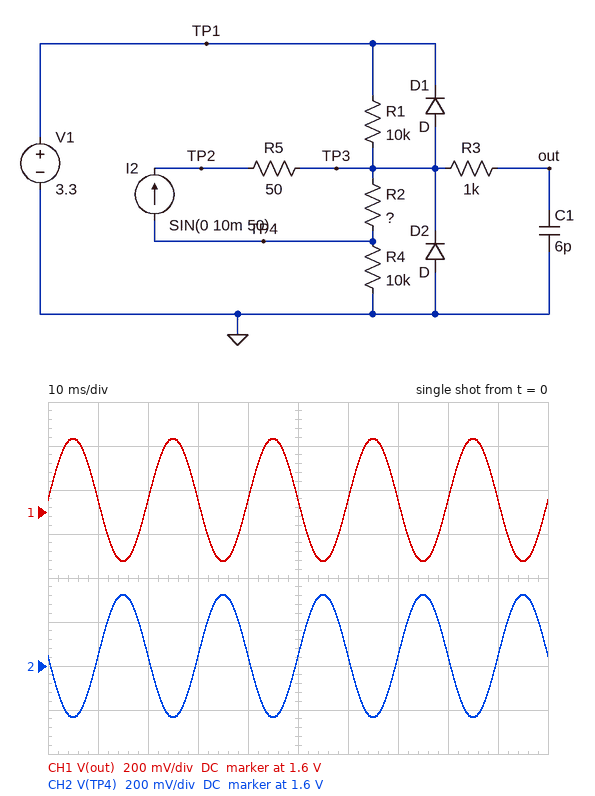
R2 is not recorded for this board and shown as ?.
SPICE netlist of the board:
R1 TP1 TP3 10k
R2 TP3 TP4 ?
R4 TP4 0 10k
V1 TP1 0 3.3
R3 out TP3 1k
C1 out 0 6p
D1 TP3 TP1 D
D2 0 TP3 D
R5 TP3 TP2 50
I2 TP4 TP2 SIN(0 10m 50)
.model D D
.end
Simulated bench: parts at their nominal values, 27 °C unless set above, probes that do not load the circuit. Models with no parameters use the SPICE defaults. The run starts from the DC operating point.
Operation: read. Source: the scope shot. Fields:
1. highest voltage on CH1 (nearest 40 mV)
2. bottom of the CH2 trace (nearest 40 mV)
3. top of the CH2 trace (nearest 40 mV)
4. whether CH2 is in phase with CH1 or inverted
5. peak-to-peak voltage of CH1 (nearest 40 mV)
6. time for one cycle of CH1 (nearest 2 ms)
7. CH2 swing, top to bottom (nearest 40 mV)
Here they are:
1.92 V
1.36 V
1.92 V
inverted
560 mV
20 ms
560 mV
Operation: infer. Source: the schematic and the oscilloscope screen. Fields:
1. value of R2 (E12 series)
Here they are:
56 Ω
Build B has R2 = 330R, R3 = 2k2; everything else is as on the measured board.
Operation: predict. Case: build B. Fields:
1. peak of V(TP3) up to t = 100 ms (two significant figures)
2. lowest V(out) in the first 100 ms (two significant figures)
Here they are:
3.3 V
54 mV
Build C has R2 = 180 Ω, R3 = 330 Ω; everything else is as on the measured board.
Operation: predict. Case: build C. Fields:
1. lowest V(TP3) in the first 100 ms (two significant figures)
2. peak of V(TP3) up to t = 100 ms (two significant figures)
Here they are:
770 mV
2.6 V
